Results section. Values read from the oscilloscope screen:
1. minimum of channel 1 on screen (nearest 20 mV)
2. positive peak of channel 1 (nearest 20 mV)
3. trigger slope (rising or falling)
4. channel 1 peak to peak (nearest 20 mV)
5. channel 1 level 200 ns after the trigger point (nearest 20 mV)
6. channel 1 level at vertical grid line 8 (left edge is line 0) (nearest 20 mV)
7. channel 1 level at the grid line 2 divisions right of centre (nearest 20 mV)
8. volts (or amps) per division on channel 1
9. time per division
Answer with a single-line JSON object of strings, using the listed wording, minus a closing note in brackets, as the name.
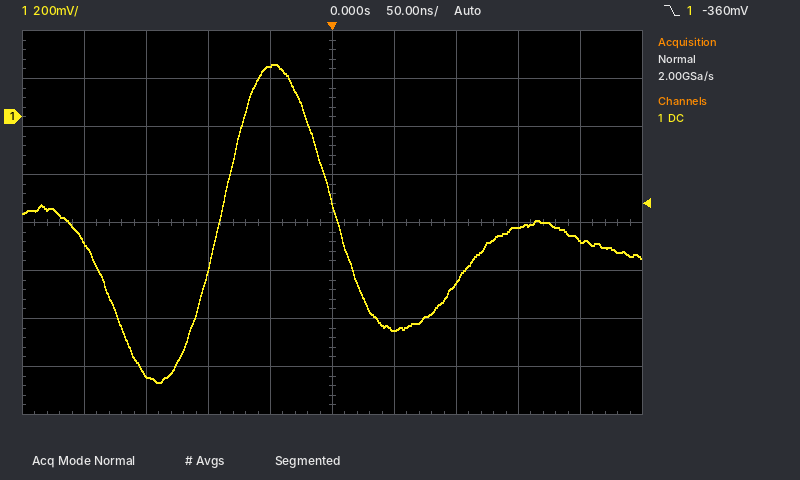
{"minimum of channel 1 on screen": "-1.10 V", "positive peak of channel 1": "220 mV", "trigger slope": "falling", "channel 1 peak to peak": "1.32 V", "channel 1 level 200 ns after the trigger point": "-520 mV", "channel 1 level at vertical grid line 8 (left edge is line 0)": "-460 mV", "channel 1 level at the grid line 2 divisions right of centre": "-700 mV", "volts (or amps) per division on channel 1": "200 mV", "time per division": "50 ns"}
